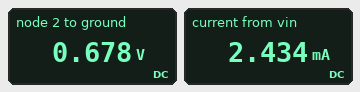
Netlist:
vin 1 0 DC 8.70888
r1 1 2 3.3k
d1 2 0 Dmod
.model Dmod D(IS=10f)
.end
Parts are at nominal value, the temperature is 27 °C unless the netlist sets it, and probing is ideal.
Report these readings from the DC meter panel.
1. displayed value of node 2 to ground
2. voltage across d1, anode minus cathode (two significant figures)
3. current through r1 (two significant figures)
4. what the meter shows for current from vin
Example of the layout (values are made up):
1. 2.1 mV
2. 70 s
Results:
1. 0.678 V
2. 680 mV
3. 2.4 mA
4. 2.434 mA
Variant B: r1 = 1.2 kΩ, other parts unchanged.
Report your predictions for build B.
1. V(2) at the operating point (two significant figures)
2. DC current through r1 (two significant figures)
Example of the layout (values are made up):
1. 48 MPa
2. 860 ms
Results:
1. 700 mV
2. 6.7 mA
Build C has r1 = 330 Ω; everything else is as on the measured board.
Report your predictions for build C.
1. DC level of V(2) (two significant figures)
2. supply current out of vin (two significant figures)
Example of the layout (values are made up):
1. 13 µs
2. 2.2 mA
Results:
1. 740 mV
2. 24 mA
